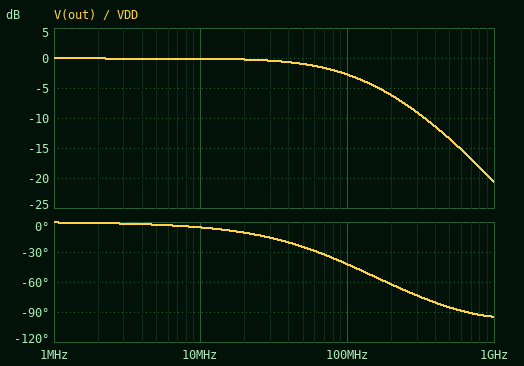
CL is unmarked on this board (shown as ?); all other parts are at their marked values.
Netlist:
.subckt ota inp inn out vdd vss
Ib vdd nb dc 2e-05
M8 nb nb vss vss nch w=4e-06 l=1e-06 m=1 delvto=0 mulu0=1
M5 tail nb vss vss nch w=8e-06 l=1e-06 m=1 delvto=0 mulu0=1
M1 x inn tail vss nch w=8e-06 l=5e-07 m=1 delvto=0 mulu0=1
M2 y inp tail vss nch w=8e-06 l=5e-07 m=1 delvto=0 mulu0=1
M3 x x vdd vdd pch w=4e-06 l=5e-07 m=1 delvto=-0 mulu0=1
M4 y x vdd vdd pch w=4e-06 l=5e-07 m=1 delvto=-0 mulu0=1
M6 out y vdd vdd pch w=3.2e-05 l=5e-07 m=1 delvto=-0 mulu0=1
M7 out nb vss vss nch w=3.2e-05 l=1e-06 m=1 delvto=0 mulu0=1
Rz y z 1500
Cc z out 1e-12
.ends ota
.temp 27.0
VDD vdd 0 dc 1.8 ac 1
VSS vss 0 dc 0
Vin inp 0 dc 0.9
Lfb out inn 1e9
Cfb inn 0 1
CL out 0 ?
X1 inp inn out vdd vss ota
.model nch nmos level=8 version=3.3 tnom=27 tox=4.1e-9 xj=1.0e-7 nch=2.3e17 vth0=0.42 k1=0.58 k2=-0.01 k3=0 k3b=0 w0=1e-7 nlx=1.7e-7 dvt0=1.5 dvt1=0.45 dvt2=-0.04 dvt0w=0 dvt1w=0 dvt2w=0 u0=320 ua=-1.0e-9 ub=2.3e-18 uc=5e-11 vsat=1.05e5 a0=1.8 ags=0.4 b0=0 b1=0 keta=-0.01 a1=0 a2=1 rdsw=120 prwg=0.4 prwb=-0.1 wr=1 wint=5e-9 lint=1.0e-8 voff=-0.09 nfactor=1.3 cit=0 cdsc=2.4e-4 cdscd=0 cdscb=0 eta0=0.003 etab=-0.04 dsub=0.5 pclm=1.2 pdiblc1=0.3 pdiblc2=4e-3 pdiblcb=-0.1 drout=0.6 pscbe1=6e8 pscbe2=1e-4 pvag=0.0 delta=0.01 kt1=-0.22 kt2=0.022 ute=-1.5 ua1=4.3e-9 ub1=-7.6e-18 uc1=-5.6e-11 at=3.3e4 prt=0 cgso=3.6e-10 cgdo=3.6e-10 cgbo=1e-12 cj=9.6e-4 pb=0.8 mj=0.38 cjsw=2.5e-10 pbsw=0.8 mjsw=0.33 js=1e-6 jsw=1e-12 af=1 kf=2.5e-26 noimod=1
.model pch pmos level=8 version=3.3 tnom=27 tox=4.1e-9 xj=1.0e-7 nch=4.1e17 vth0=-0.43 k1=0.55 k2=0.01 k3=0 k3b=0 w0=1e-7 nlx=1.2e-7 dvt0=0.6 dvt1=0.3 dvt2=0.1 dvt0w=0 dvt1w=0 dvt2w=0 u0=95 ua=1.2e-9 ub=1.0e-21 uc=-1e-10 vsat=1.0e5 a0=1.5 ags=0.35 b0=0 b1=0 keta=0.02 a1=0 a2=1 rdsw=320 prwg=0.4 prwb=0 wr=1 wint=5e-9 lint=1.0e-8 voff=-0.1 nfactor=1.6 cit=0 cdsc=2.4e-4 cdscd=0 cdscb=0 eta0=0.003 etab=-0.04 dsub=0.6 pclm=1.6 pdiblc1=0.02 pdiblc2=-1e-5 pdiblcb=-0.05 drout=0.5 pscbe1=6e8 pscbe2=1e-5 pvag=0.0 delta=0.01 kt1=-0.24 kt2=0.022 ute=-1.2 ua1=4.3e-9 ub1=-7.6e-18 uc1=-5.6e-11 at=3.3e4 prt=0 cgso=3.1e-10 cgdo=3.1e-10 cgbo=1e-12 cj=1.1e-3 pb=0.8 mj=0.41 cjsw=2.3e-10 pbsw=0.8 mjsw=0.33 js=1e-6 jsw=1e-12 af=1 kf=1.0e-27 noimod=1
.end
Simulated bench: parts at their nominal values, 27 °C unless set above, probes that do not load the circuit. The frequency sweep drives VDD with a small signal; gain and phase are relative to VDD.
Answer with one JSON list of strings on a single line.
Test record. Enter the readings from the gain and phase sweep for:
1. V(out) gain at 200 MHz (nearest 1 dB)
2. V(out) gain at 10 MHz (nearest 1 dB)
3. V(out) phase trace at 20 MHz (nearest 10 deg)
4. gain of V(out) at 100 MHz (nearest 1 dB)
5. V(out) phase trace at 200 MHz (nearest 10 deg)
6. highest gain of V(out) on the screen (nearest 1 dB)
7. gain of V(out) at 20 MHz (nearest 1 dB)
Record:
["-6 dB", "0 dB", "-10 deg", "-3 dB", "-60 deg", "0 dB", "0 dB"]
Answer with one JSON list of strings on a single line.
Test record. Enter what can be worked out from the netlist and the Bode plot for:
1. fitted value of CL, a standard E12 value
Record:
["1.2 pF"]
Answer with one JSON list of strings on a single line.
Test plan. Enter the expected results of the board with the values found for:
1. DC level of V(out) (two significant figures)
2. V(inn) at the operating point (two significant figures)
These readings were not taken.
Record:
["900 mV", "900 mV"]
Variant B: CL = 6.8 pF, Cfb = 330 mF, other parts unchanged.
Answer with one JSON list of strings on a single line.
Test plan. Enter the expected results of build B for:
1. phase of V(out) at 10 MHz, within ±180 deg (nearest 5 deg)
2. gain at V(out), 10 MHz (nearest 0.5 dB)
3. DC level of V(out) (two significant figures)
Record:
["-25 deg", "-1.0 dB", "900 mV"]
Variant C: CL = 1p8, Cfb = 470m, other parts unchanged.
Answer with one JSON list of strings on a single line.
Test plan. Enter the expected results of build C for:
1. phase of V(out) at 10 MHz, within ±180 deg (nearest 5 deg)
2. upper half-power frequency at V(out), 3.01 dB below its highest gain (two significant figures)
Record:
["-10 deg", "74 MHz"]
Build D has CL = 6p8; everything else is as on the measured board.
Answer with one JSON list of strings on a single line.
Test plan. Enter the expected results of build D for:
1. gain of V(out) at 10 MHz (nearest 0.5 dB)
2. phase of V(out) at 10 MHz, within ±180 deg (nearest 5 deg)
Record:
["-1.0 dB", "-25 deg"]
